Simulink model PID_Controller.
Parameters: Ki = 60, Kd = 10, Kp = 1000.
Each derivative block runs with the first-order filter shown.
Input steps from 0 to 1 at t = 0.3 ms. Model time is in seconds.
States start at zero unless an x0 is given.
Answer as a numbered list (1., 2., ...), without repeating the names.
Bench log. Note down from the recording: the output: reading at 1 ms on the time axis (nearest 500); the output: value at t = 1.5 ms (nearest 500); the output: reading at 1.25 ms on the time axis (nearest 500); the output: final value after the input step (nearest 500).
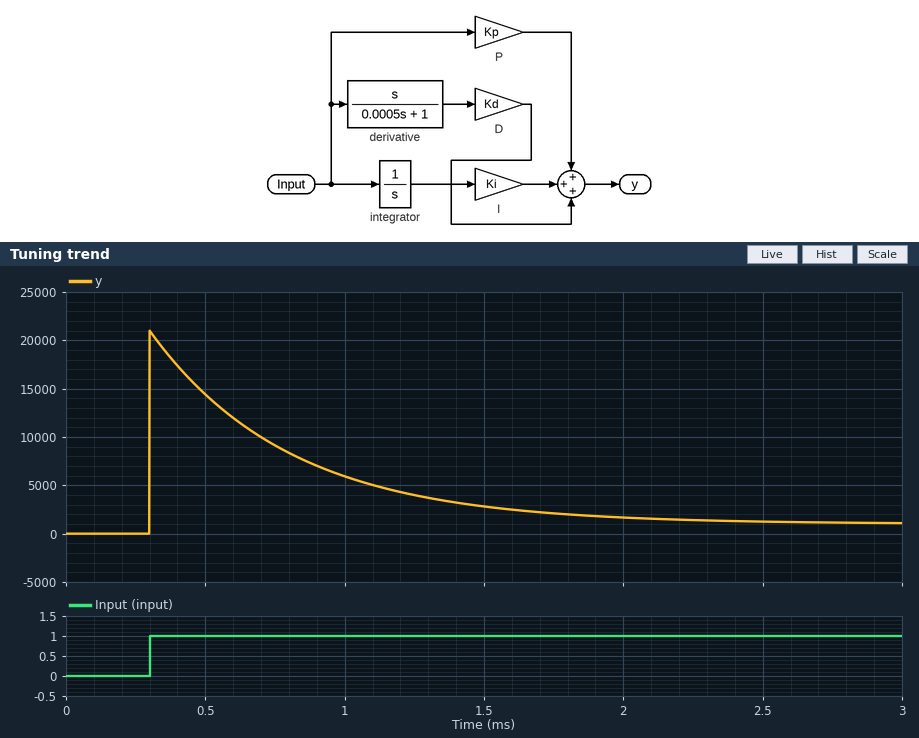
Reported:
1. 6000
2. 3000
3. 4000
4. 1000
